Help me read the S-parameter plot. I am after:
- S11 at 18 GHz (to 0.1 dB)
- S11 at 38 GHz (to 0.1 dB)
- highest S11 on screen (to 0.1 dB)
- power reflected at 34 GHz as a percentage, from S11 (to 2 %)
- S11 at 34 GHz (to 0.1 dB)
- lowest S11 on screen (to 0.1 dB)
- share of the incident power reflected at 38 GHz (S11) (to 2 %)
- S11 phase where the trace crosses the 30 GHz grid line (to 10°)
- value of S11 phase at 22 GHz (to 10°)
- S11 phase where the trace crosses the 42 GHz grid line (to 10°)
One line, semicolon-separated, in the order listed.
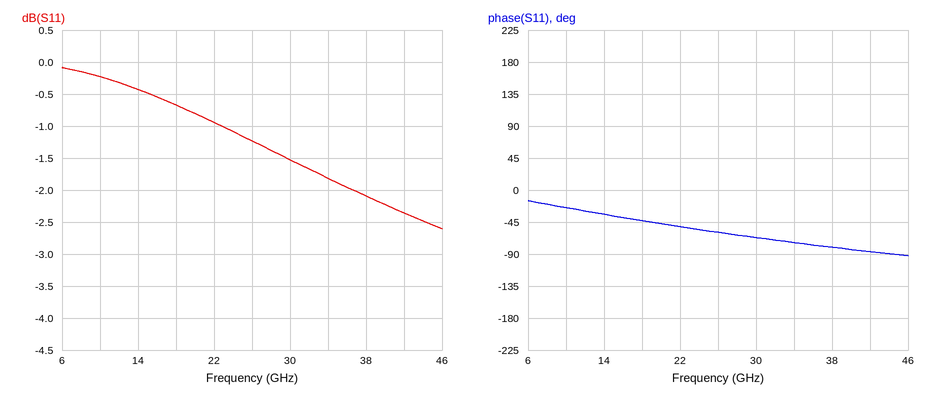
-0.7 dB; -2.1 dB; -0.1 dB; 66 %; -1.8 dB; -2.6 dB; 62 %; -70°; -50°; -90°
